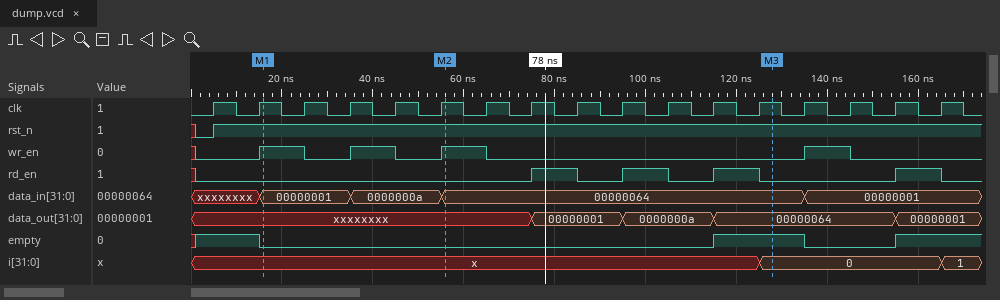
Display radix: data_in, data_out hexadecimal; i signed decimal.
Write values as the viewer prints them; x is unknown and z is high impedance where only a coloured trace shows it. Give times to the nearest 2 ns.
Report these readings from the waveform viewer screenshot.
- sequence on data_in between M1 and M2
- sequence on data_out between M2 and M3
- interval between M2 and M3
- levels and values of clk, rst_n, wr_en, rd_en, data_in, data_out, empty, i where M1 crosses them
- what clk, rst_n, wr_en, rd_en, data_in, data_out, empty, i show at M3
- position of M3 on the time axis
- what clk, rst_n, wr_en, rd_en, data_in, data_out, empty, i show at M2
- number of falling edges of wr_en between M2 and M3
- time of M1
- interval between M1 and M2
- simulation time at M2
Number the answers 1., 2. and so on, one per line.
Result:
1. 00000001, 0000000a, 00000064
2. xxxxxxxx, 00000001, 0000000a, 00000064
3. 72 ns
4. clk=1, rst_n=1, wr_en=1, rd_en=0, data_in=00000001, data_out=xxxxxxxx, empty=0, i=x
5. clk=1, rst_n=1, wr_en=0, rd_en=0, data_in=00000064, data_out=00000064, empty=1, i=0
6. 128 ns
7. clk=1, rst_n=1, wr_en=1, rd_en=0, data_in=00000064, data_out=xxxxxxxx, empty=0, i=x
8. 1
9. 16 ns
10. 40 ns
11. 56 ns
